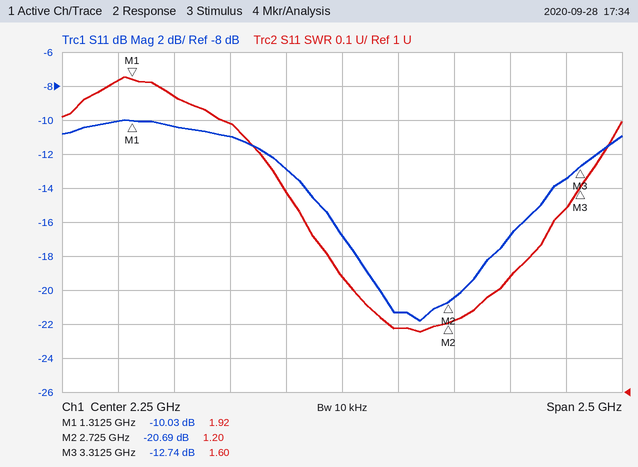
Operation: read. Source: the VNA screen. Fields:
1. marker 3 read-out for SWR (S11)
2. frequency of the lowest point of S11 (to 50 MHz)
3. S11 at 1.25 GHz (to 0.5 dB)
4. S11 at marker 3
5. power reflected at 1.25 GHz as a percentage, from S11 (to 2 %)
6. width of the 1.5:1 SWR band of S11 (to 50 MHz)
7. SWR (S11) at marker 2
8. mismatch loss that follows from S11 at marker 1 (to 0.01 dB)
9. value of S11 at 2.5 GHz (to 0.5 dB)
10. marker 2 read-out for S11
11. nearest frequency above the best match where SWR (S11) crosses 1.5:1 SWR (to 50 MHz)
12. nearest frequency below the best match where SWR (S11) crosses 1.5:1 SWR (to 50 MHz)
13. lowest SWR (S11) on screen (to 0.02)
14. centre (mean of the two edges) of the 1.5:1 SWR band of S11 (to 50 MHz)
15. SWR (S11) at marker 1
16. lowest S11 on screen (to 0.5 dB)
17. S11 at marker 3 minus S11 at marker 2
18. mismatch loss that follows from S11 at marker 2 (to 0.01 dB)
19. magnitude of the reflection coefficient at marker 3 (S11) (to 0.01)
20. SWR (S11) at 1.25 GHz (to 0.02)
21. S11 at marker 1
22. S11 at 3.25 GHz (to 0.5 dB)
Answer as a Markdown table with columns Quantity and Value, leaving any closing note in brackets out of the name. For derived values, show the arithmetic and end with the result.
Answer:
| Quantity | Value |
|---|---|
| marker 3 read-out for SWR | 1.60 |
| frequency of the lowest point of S11 | 2.60 GHz |
| S11 at 1.25 GHz | -10.0 dB |
| S11 at marker 3 | -12.74 dB |
| power reflected at 1.25 GHz as a percentage, from S11 | 10^(-10/10) ≈ 10 % |
| width of the 1.5:1 SWR band of S11 | 3.20 GHz − 2.10 GHz = 1.10 GHz |
| SWR (S11) at marker 2 | 1.20 |
| mismatch loss that follows from S11 at marker 1 | −10 log10(1 − 10^(-10.03/10)) ≈ 0.45 dB |
| value of S11 at 2.5 GHz | -21.5 dB |
| marker 2 read-out for S11 | -20.69 dB |
| nearest frequency above the best match where SWR (S11) crosses 1.5:1 SWR | 3.20 GHz |
| nearest frequency below the best match where SWR (S11) crosses 1.5:1 SWR | 2.10 GHz |
| lowest SWR (S11) on screen | 1.18 |
| centre (mean of the two edges) of the 1.5:1 SWR band of S11 | 2.65 GHz |
| SWR (S11) at marker 1 | 1.92 |
| lowest S11 on screen | -22.0 dB |
| S11 at marker 3 minus S11 at marker 2 | -12.74 − (-20.69) = 7.95 dB |
| mismatch loss that follows from S11 at marker 2 | −10 log10(1 − 10^(-20.69/10)) ≈ 0.04 dB |
| magnitude of the reflection coefficient at marker 3 (S11) | 10^(-12.74/20) ≈ 0.23 |
| SWR (S11) at 1.25 GHz | 1.92 |
| S11 at marker 1 | -10.03 dB |
| S11 at 3.25 GHz | -13.5 dB |
